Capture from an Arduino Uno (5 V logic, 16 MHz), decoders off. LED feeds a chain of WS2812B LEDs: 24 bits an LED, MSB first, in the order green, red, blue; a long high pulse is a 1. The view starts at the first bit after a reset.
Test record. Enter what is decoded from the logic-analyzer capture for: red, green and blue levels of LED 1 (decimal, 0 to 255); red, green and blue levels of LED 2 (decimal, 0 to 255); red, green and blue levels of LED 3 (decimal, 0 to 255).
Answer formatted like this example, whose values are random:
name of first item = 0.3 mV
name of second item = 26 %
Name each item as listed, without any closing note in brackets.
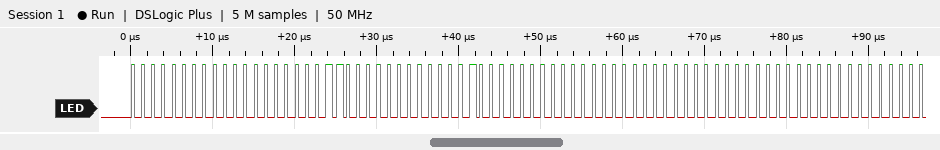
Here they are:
red, green and blue levels of LED 1 = 0, 0, 24
red, green and blue levels of LED 2 = 64, 0, 0
red, green and blue levels of LED 3 = 0, 0, 0
